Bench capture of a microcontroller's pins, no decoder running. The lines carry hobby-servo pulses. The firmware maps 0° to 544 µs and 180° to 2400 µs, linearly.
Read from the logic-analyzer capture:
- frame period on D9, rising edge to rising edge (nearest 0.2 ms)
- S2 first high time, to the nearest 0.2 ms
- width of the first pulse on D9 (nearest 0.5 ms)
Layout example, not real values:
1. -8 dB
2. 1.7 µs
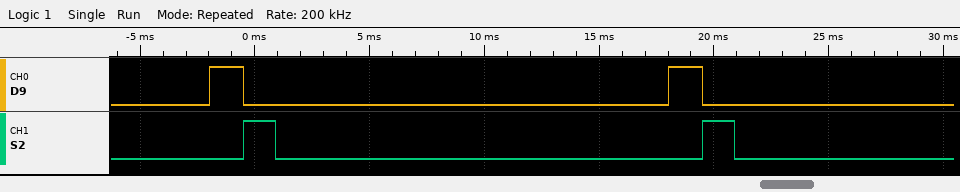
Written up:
1. 20.0 ms
2. 1.4 ms
3. 1.5 ms
